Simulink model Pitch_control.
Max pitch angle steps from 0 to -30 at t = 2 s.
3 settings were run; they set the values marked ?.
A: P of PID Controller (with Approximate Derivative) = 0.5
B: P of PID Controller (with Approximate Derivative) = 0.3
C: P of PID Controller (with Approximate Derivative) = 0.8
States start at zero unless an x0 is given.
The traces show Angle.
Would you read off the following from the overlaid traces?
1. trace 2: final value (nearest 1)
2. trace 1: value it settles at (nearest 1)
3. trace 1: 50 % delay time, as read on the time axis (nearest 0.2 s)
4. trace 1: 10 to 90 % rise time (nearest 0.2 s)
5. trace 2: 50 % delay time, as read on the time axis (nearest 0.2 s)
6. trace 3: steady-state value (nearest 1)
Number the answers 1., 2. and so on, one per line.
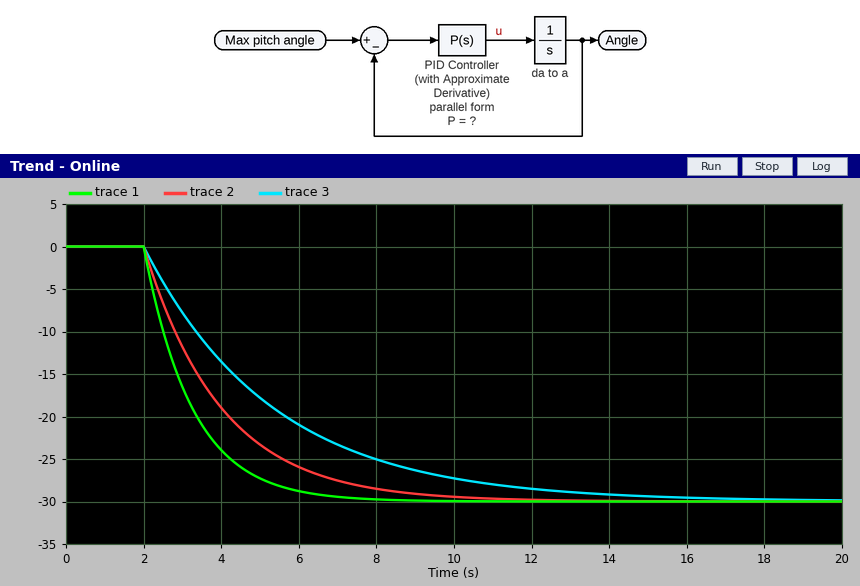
1. -30
2. -30
3. 2.8 s
4. 2.8 s
5. 3.4 s
6. -30
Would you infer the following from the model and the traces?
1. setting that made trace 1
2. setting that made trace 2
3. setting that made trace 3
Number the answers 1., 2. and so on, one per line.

1. C
2. A
3. B
